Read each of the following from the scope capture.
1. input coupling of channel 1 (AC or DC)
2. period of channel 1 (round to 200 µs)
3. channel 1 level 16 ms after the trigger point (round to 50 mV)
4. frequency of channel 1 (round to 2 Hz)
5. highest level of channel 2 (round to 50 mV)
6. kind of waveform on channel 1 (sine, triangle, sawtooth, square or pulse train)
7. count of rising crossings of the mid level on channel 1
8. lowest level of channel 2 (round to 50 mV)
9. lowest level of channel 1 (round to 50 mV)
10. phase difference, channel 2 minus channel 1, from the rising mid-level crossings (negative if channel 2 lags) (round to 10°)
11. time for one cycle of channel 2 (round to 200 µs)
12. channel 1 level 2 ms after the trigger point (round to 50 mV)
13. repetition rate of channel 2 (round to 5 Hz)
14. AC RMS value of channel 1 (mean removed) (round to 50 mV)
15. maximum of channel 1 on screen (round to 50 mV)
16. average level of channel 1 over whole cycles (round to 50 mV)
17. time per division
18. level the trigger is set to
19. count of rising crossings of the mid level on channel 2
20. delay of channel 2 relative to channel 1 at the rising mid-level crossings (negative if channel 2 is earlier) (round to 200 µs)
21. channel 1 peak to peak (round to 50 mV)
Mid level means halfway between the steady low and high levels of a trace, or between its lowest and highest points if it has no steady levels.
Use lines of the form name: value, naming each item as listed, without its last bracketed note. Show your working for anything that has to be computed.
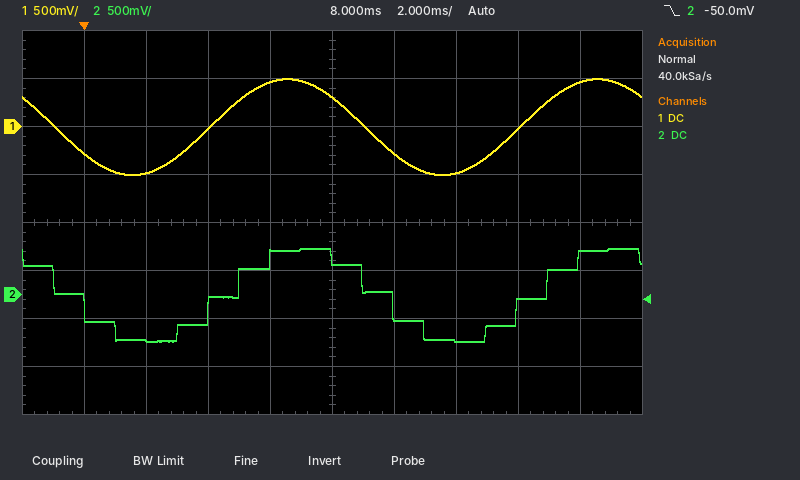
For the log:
input coupling of channel 1: DC
period of channel 1: 10.0 ms
channel 1 level 16 ms after the trigger point: 450 mV
frequency of channel 1: 1 / 10.0 ms ≈ 100 Hz
highest level of channel 2: 500 mV
kind of waveform on channel 1: sine
count of rising crossings of the mid level on channel 1: 2
lowest level of channel 2: -500 mV
lowest level of channel 1: -500 mV
phase difference, channel 2 minus channel 1, from the rising mid-level crossings (negative if channel 2 lags): −360° × (+800 µs) / 10.0 ms ≈ -28.8°, so -30° to the nearest 10°
time for one cycle of channel 2: 10.0 ms
channel 1 level 2 ms after the trigger point: -500 mV
repetition rate of channel 2: 1 / 10.0 ms ≈ 100 Hz
AC RMS value of channel 1 (mean removed): 1.00 V / (2√2) ≈ 354 mV, so 350 mV to the nearest 50 mV
maximum of channel 1 on screen: 500 mV
average level of channel 1 over whole cycles: (500 mV + (-500 mV)) / 2 ≈ 0 mV
time per division: 2 ms
level the trigger is set to: -50.0 mV
count of rising crossings of the mid level on channel 2: 2
delay of channel 2 relative to channel 1 at the rising mid-level crossings (negative if channel 2 is earlier): +800 µs
channel 1 peak to peak: 500 mV − (-500 mV) = 1.00 V
